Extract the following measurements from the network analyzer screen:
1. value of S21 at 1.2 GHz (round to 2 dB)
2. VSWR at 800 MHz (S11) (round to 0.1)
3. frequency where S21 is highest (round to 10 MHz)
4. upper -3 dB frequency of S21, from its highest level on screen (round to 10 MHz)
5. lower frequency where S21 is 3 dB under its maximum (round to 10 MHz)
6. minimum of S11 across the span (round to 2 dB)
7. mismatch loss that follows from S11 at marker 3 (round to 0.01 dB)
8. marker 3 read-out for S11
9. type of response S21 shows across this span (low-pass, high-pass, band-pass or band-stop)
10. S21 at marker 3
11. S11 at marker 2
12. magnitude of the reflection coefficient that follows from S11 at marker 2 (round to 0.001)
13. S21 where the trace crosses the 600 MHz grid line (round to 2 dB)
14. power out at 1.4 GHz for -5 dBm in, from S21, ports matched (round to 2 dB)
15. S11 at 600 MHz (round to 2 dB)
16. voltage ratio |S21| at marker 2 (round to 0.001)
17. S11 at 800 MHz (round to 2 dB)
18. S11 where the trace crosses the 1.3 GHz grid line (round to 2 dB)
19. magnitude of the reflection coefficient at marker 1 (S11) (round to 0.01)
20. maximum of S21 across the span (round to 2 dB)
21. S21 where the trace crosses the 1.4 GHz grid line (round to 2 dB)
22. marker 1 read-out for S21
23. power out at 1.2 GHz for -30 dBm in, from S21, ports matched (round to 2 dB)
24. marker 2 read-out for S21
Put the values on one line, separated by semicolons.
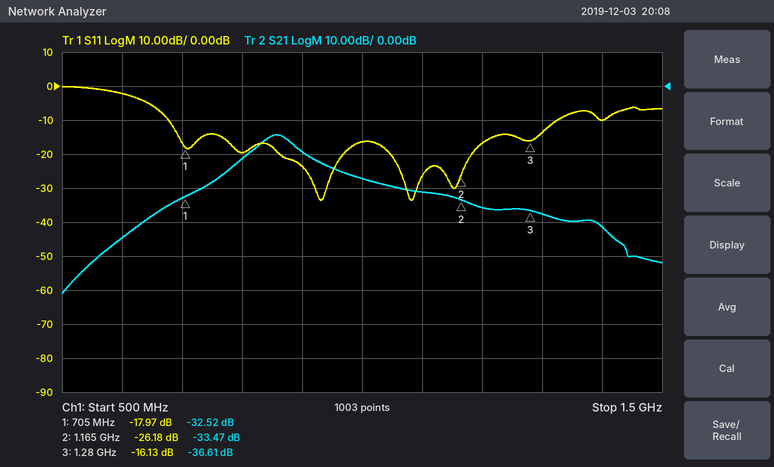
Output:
-36 dB; 1.2; 860 MHz; 890 MHz; 830 MHz; -34 dB; 0.11 dB; -16.13 dB; band-pass; -36.61 dB; -26.18 dB; 0.049; -44 dB; -46 dBm; -2 dB; 0.021; -20 dB; -14 dB; 0.13; -14 dB; -42 dB; -32.52 dB; -66 dBm; -33.47 dB
